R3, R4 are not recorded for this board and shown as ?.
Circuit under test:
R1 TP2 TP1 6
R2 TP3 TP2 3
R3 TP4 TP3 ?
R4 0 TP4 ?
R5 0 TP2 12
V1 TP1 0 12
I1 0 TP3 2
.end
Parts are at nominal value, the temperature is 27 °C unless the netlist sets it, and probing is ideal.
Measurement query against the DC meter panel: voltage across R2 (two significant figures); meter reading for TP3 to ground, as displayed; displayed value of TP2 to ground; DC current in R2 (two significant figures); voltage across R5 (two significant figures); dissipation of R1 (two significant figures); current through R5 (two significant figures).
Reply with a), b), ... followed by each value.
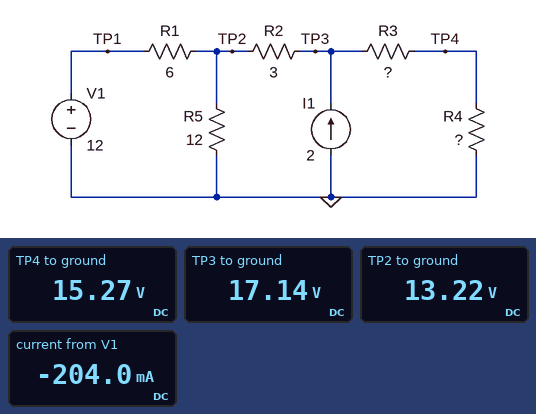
a) 3.9 V
b) 17.14 V
c) 13.22 V
d) 1.3 A
e) 13 V
f) 250 mW
g) 1.1 A
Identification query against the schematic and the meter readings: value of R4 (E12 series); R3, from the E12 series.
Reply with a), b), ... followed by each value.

a) 22 Ω
b) 2.7 Ω
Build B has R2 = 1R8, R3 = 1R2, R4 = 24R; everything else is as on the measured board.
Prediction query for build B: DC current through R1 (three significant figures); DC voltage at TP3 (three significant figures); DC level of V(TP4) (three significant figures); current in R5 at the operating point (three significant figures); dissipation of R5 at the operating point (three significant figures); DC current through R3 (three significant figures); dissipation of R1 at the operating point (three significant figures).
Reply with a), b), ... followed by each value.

a) 245 mA
b) 15.9 V
c) 15.2 V
d) 1.12 A
e) 15.1 W
f) 632 mA
g) 361 mW
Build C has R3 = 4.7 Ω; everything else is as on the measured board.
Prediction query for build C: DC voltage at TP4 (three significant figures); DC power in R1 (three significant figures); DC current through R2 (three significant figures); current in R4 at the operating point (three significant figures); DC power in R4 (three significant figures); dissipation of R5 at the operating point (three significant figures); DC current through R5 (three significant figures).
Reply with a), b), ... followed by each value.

a) 14.4 V
b) 321 mW
c) 1.35 A
d) 653 mA
e) 9.38 W
f) 14.9 W
g) 1.12 A
